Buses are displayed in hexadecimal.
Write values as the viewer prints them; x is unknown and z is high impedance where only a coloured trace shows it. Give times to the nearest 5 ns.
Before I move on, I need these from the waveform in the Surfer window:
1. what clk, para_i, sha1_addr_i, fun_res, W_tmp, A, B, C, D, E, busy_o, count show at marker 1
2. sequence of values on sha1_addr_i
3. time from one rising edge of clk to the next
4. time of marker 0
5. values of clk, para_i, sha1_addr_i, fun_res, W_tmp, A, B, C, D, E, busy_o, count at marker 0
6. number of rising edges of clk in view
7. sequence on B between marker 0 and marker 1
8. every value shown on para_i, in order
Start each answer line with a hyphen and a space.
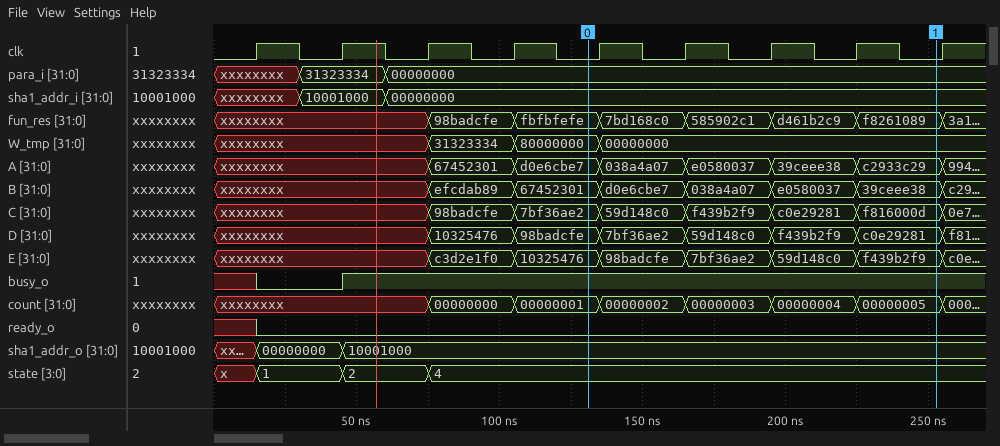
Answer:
- clk=0, para_i=00000000, sha1_addr_i=00000000, fun_res=f8261089, W_tmp=00000000, A=c2933c29, B=39ceee38, C=f816000d, D=c0e29281, E=f439b2f9, busy_o=1, count=00000005
- xxxxxxxx, 10001000, 00000000
- 30 ns
- 130 ns
- clk=0, para_i=00000000, sha1_addr_i=00000000, fun_res=fbfbfefe, W_tmp=80000000, A=d0e6cbe7, B=67452301, C=7bf36ae2, D=98badcfe, E=10325476, busy_o=1, count=00000001
- 9
- 67452301, d0e6cbe7, 038a4a07, e0580037, 39ceee38
- xxxxxxxx, 31323334, 00000000
